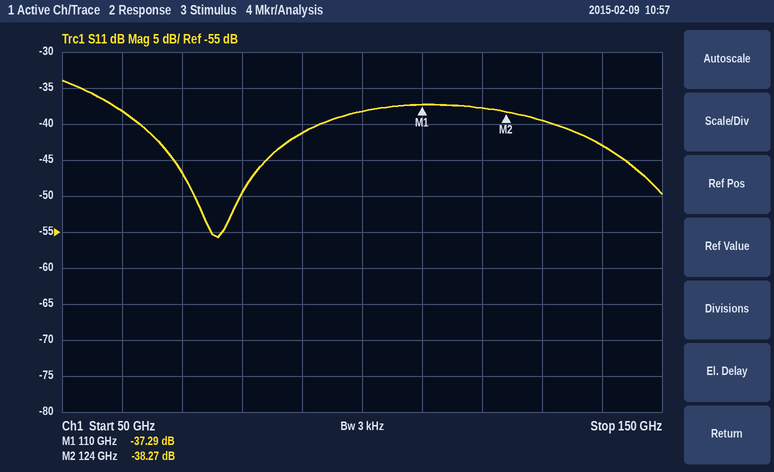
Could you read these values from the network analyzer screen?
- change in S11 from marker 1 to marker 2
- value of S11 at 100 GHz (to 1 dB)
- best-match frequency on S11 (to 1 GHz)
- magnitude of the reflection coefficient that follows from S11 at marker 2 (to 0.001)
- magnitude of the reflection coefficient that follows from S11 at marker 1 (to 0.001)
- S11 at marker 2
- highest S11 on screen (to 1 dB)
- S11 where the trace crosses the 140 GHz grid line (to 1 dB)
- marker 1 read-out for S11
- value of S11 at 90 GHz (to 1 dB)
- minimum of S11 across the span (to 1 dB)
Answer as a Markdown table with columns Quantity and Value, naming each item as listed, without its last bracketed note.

| Quantity | Value |
|---|---|
| change in S11 from marker 1 to marker 2 | -0.98 dB |
| value of S11 at 100 GHz | -38 dB |
| best-match frequency on S11 | 76 GHz |
| magnitude of the reflection coefficient that follows from S11 at marker 2 | 0.012 |
| magnitude of the reflection coefficient that follows from S11 at marker 1 | 0.014 |
| S11 at marker 2 | -38.27 dB |
| highest S11 on screen | -34 dB |
| S11 where the trace crosses the 140 GHz grid line | -43 dB |
| marker 1 read-out for S11 | -37.29 dB |
| value of S11 at 90 GHz | -41 dB |
| minimum of S11 across the span | -56 dB |
